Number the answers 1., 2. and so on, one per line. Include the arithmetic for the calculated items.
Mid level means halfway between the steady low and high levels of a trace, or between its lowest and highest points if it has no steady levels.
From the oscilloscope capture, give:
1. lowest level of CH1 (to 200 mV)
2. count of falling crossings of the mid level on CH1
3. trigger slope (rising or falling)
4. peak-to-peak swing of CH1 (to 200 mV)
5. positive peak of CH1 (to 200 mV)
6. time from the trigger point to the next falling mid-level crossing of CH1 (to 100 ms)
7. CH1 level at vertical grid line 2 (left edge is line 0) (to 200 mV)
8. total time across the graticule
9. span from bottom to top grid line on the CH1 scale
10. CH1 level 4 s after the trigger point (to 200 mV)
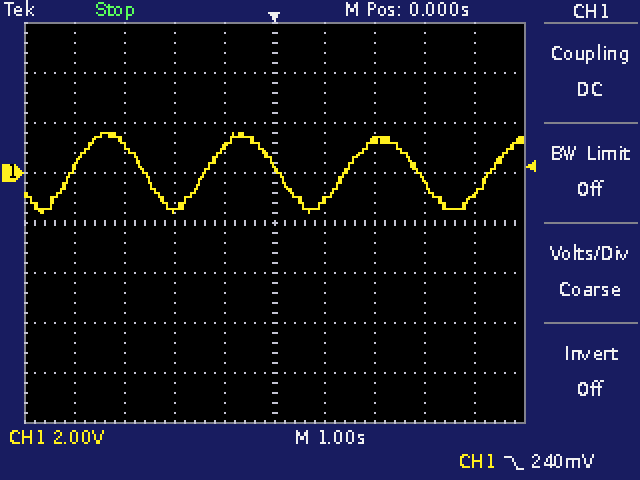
1. -1.6 V
2. 3
3. falling
4. 1.6 V − (-1.6 V) = 3.2 V
5. 1.6 V
6. 100 ms
7. 1.2 V
8. 10 s
9. 16 V
10. -800 mV
